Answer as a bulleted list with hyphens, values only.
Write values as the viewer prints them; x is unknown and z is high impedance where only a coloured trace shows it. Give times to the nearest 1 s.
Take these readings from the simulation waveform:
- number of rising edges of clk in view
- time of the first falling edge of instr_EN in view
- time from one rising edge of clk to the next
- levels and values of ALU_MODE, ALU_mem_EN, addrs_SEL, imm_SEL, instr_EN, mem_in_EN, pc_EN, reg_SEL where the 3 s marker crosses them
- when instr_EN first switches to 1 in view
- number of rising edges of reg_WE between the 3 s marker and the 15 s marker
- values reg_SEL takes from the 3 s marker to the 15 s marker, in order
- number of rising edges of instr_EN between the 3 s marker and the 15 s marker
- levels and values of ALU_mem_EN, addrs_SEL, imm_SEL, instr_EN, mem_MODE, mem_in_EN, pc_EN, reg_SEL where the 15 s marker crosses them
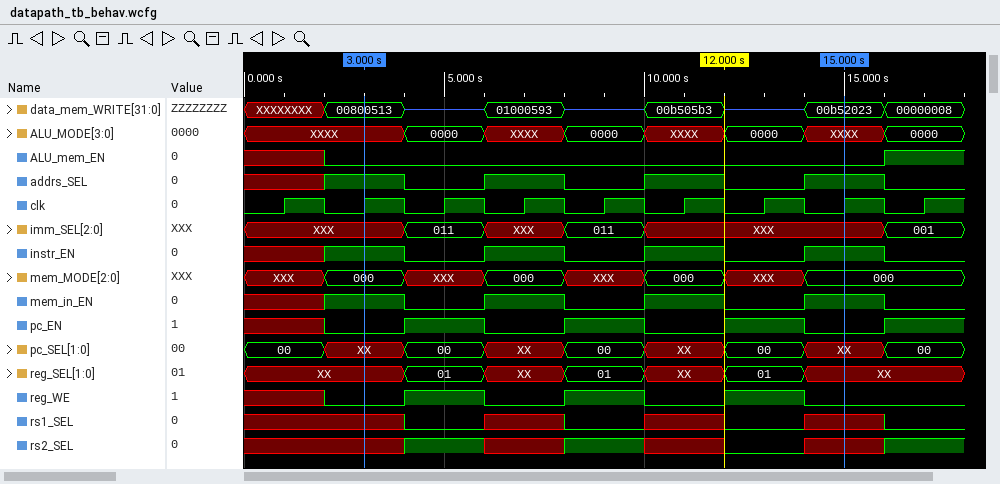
- 9
- 4 s
- 2 s
- ALU_MODE=XXXX, ALU_mem_EN=0, addrs_SEL=1, imm_SEL=XXX, instr_EN=1, mem_in_EN=1, pc_EN=0, reg_SEL=XX
- 2 s
- 3
- XX, 01, XX, 01, XX, 01, XX
- 3
- ALU_mem_EN=0, addrs_SEL=1, imm_SEL=XXX, instr_EN=1, mem_MODE=000, mem_in_EN=1, pc_EN=0, reg_SEL=XX
